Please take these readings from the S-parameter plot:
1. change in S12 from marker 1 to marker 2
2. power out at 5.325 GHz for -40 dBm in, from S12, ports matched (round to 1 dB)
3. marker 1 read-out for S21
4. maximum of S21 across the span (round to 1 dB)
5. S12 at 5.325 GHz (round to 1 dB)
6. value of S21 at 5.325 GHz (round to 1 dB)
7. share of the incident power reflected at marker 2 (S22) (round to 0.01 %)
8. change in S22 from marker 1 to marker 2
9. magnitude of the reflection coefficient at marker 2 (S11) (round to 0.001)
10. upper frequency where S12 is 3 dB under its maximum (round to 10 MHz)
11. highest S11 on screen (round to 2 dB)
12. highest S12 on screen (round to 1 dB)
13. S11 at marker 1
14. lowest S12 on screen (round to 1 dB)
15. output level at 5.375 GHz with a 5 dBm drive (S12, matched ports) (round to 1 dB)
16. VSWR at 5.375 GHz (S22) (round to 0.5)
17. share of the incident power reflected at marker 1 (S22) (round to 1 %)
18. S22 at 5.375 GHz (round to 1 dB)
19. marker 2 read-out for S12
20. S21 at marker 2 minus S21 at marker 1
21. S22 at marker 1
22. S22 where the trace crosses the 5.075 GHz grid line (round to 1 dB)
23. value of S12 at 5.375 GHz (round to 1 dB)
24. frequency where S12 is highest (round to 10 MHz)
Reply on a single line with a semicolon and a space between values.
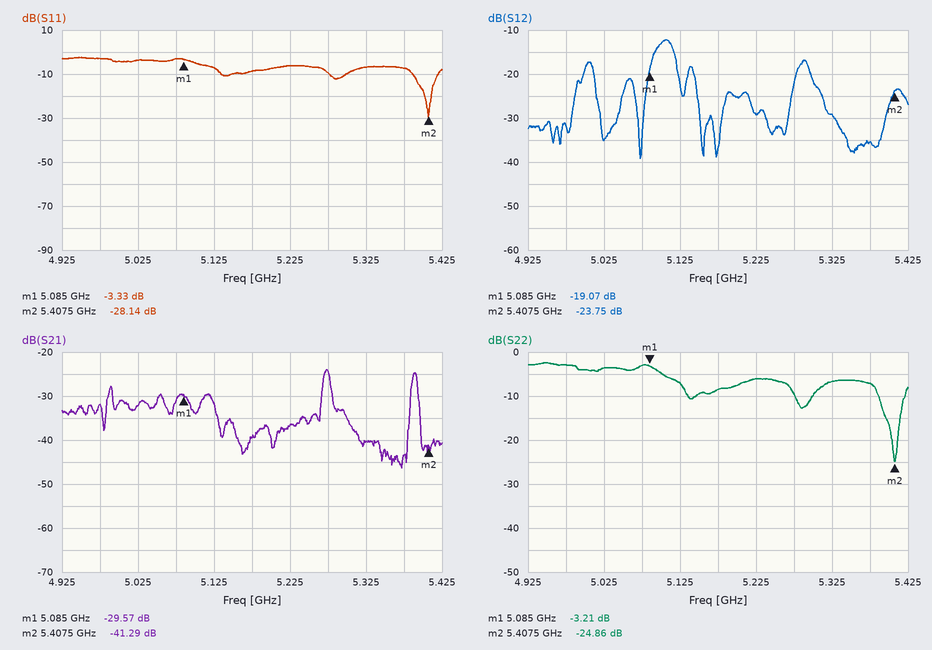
-4.68 dB; -69 dBm; -29.57 dB; -24 dB; -29 dB; -40 dB; 0.33 %; -21.65 dB; 0.039; 5.12 GHz; -2 dB; -12 dB; -3.33 dB; -39 dB; -30 dBm; 2.5; 48 %; -7 dB; -23.75 dB; -11.72 dB; -3.21 dB; -3 dB; -35 dB; 5.11 GHz
